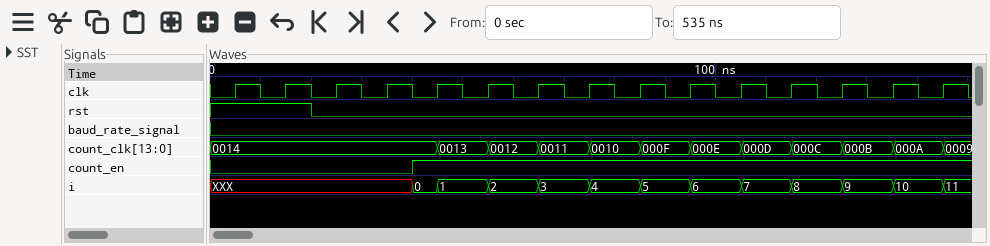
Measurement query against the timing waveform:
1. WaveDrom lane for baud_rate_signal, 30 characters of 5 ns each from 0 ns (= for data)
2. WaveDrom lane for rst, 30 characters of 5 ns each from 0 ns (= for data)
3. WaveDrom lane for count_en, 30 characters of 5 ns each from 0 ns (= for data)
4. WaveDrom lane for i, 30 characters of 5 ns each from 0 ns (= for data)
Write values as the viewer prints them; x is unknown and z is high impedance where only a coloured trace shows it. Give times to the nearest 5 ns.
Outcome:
{name: 'baud_rate_signal', wave: '0.............................'}
{name: 'rst', wave: '1...0.........................'}
{name: 'count_en', wave: '0.......1.....................'}
{name: 'i', wave: 'x.......==.=.=.=.=.=.=.=.=.=.=', data: '0 1 2 3 4 5 6 7 8 9 10 11'}
